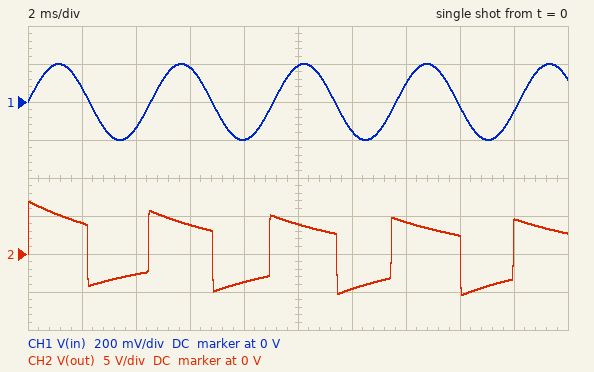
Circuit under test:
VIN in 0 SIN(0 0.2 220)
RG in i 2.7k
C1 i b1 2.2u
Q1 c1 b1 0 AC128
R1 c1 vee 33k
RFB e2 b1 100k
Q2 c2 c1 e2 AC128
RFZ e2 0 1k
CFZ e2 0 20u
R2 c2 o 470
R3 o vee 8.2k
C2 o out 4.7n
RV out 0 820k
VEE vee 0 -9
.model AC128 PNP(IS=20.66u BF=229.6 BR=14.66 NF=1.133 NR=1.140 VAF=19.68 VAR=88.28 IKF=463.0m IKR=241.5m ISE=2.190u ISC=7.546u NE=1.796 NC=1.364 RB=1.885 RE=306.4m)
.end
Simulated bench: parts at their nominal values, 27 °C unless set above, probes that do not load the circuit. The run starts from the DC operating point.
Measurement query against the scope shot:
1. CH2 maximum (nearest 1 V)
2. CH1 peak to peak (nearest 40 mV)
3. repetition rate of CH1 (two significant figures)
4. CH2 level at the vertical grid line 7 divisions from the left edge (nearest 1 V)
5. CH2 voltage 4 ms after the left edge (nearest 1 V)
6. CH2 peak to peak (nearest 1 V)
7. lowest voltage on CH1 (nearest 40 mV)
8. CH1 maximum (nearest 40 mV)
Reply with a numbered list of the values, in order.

1. 7 V
2. 400 mV
3. 220 Hz
4. 4 V
5. -3 V
6. 12 V
7. -200 mV
8. 200 mV
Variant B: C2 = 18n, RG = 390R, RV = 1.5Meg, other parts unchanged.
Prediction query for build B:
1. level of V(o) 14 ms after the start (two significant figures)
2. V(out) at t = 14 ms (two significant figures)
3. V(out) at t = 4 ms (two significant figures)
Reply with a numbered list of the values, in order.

1. -980 mV
2. 5.0 V
3. -1.7 V
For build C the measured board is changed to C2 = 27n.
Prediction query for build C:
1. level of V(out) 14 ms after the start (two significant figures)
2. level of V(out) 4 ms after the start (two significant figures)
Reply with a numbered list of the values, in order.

1. 5.3 V
2. -1.8 V
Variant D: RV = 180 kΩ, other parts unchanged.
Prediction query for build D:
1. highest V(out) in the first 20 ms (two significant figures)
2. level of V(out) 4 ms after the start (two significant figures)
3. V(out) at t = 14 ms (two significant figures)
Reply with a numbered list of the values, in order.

1. 7.3 V
2. -970 mV
3. 3.8 V
